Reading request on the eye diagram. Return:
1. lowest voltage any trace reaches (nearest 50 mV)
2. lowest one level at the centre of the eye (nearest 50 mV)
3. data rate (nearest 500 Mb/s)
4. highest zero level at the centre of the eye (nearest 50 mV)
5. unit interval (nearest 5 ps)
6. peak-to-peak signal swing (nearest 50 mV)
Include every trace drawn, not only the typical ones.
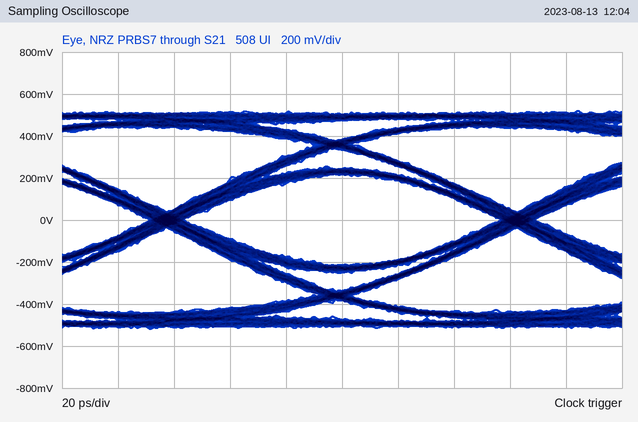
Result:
-500 mV
200 mV
8.0 Gb/s
-200 mV
125 ps
1.05 V
